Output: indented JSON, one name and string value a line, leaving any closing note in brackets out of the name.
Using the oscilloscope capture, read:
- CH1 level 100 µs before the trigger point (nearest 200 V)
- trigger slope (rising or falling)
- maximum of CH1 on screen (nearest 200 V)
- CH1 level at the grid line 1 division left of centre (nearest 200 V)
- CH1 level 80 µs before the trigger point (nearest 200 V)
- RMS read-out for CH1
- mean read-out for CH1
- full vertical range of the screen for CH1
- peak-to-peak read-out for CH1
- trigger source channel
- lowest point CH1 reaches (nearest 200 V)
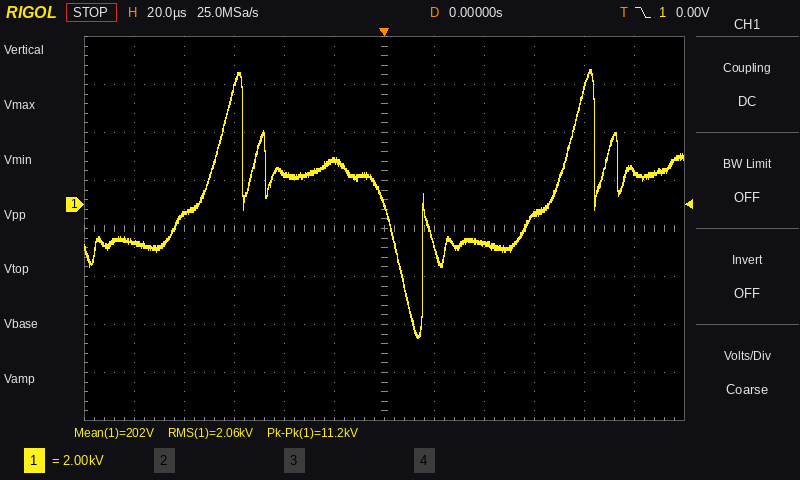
{
  "CH1 level 100 µs before the trigger point": "-1.6 kV",
  "trigger slope": "falling",
  "maximum of CH1 on screen": "5.6 kV",
  "CH1 level at the grid line 1 division left of centre": "1.8 kV",
  "CH1 level 80 µs before the trigger point": "-400 V",
  "RMS read-out for CH1": "2.06 kV",
  "mean read-out for CH1": "202 V",
  "full vertical range of the screen for CH1": "16 kV",
  "peak-to-peak read-out for CH1": "11.2 kV",
  "trigger source channel": "CH1",
  "lowest point CH1 reaches": "-5.6 kV"
}
